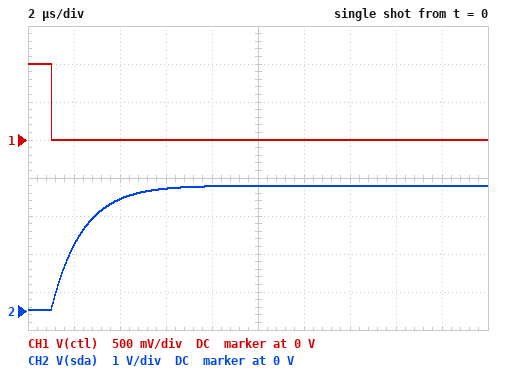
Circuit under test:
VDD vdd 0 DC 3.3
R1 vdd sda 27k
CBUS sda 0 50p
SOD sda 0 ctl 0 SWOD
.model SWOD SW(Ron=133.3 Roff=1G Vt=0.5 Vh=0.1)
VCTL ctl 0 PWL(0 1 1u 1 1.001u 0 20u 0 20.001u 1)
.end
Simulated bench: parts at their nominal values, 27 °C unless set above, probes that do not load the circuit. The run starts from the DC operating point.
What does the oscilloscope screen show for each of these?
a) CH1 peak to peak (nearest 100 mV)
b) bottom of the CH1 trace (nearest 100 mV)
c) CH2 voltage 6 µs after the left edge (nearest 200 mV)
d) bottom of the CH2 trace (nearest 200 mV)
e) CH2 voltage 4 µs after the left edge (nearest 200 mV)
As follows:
1.0 V
0 V
3.2 V
0 V
3.0 V
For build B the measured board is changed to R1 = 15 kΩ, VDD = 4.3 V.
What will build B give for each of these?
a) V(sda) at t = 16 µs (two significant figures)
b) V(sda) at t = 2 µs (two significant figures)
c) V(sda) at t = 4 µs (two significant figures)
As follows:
4.3 V
3.2 V
4.2 V
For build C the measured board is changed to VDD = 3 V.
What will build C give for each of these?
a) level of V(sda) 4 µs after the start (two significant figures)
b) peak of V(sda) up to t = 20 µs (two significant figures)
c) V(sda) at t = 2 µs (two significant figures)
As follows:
2.7 V
3.0 V
1.6 V
